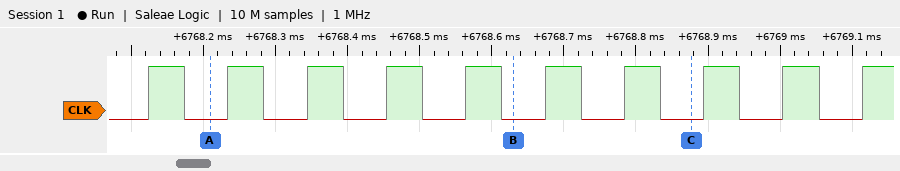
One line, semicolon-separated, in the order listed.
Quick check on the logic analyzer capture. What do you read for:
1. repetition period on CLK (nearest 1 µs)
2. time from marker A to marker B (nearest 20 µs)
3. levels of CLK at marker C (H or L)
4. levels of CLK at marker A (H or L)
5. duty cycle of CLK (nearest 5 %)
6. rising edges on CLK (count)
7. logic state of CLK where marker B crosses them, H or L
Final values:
110 µs; 420 µs; CLK=L; CLK=L; 45 %; 10; CLK=L
